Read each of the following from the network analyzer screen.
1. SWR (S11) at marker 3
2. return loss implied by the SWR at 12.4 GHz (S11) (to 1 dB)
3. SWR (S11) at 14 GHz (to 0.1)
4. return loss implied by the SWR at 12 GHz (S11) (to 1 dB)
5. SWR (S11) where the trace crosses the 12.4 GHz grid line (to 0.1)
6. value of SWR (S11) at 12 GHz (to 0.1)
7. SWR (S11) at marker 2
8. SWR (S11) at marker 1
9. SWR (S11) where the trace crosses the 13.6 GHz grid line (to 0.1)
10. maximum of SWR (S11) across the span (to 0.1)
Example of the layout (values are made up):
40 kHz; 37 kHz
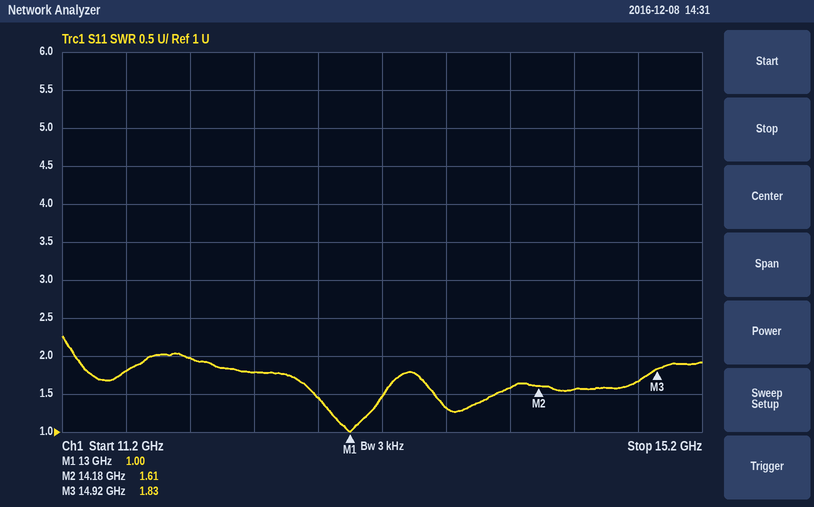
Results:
1.83; 11 dB; 1.6; 10 dB; 1.8; 2.0; 1.61; 1.00; 1.3; 2.3
